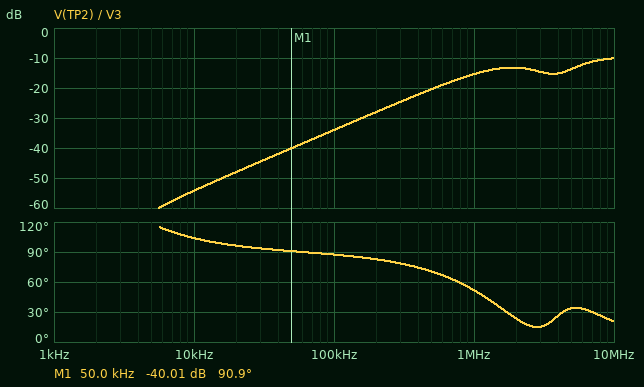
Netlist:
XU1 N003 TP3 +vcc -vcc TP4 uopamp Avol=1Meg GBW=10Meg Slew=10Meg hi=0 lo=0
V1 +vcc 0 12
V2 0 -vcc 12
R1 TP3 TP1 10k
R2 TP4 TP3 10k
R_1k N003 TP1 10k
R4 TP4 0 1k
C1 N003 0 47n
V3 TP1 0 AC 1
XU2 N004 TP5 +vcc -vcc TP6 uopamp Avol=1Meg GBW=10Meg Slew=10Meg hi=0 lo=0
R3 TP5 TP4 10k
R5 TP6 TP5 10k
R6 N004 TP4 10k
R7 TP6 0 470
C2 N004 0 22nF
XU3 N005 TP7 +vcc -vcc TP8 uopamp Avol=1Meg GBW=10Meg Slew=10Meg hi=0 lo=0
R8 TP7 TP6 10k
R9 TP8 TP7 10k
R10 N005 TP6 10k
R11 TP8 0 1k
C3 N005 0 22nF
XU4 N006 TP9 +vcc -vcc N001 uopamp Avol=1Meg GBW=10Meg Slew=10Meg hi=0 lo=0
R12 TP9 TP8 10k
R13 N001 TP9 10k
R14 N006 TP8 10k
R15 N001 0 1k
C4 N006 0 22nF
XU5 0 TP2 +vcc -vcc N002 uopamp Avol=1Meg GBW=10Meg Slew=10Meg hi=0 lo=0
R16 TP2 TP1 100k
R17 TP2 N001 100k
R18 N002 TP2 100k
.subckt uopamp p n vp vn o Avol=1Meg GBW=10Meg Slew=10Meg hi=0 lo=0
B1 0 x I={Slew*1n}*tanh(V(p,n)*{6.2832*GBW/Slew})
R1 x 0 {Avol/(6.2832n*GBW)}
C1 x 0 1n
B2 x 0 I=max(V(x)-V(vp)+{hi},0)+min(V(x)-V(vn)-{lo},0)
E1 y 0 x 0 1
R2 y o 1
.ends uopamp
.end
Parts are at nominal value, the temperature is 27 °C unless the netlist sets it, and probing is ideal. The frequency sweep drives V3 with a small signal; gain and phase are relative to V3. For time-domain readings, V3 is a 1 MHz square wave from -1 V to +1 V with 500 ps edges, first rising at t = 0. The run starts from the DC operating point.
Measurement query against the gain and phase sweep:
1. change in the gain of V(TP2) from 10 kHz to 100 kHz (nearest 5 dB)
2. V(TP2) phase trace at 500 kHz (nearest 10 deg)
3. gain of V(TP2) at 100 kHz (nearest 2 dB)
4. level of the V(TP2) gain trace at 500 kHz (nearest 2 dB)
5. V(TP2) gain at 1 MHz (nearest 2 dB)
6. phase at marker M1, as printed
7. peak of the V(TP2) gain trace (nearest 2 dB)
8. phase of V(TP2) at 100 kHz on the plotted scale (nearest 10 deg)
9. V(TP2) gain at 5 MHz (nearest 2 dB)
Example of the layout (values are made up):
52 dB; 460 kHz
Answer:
20 dB; 70 deg; -34 dB; -20 dB; -16 dB; 90.9 deg; -10 dB; 90 deg; -14 dB
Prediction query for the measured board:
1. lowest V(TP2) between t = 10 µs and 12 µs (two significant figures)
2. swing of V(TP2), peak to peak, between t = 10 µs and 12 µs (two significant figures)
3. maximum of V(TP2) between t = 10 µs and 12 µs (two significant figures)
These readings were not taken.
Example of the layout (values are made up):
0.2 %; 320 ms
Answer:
-650 mV; 1.3 V; 650 mV
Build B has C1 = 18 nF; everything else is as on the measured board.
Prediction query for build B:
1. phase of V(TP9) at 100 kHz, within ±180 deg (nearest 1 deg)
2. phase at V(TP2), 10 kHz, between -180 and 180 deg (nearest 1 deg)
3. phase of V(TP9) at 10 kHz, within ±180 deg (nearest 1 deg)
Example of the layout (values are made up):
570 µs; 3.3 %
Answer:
-93 deg; 107 deg; 120 deg
